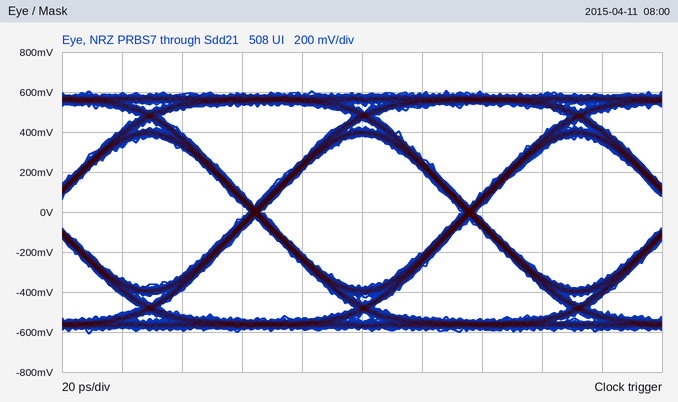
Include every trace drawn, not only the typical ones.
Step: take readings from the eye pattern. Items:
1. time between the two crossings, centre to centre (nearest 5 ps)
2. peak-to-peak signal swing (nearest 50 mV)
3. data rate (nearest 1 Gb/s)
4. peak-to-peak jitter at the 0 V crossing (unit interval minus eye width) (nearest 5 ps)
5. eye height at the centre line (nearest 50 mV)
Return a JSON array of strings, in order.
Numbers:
["70 ps", "1.20 V", "14 Gb/s", "5 ps", "750 mV"]
